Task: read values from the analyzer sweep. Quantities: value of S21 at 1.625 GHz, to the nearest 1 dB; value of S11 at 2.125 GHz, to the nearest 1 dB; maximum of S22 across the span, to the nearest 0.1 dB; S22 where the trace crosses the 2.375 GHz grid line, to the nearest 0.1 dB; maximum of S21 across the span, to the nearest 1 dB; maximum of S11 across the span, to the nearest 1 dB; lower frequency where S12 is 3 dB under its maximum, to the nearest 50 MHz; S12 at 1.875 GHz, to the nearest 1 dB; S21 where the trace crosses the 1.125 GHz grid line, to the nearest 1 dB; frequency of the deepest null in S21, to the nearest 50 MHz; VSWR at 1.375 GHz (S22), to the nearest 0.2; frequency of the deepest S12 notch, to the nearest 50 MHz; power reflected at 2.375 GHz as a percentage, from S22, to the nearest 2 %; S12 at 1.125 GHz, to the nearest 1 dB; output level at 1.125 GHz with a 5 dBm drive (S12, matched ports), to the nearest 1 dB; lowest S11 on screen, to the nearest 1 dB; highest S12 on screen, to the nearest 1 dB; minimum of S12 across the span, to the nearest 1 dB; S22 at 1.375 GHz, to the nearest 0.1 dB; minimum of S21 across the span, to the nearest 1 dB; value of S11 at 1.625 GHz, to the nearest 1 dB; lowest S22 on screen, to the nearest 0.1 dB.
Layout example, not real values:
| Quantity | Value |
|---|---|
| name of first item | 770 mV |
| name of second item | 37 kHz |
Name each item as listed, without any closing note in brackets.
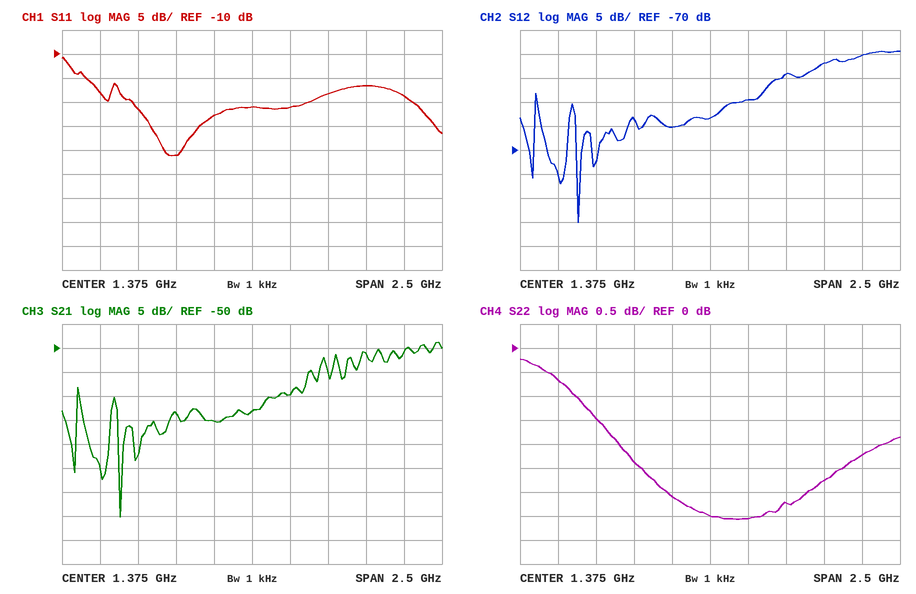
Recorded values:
| Quantity | Value |
|---|---|
| value of S21 at 1.625 GHz, to the nearest 1 dB | -60 dB |
| value of S11 at 2.125 GHz, to the nearest 1 dB | -17 dB |
| maximum of S22 across the span, to the nearest 0.1 dB | -0.2 dB |
| S22 where the trace crosses the 2.375 GHz grid line, to the nearest 0.1 dB | -2.2 dB |
| maximum of S21 across the span, to the nearest 1 dB | -49 dB |
| maximum of S11 across the span, to the nearest 1 dB | -11 dB |
| lower frequency where S12 is 3 dB under its maximum, to the nearest 50 MHz | 2.10 GHz |
| S12 at 1.875 GHz, to the nearest 1 dB | -54 dB |
| S21 where the trace crosses the 1.125 GHz grid line, to the nearest 1 dB | -65 dB |
| frequency of the deepest null in S21, to the nearest 50 MHz | 500 MHz |
| VSWR at 1.375 GHz (S22), to the nearest 0.2 | 5.0 |
| frequency of the deepest S12 notch, to the nearest 50 MHz | 500 MHz |
| power reflected at 2.375 GHz as a percentage, from S22, to the nearest 2 % | 60 % |
| S12 at 1.125 GHz, to the nearest 1 dB | -65 dB |
| output level at 1.125 GHz with a 5 dBm drive (S12, matched ports), to the nearest 1 dB | -60 dBm |
| lowest S11 on screen, to the nearest 1 dB | -31 dB |
| highest S12 on screen, to the nearest 1 dB | -49 dB |
| minimum of S12 across the span, to the nearest 1 dB | -85 dB |
| S22 at 1.375 GHz, to the nearest 0.1 dB | -3.5 dB |
| minimum of S21 across the span, to the nearest 1 dB | -85 dB |
| value of S11 at 1.625 GHz, to the nearest 1 dB | -21 dB |
| lowest S22 on screen, to the nearest 0.1 dB | -3.6 dB |
